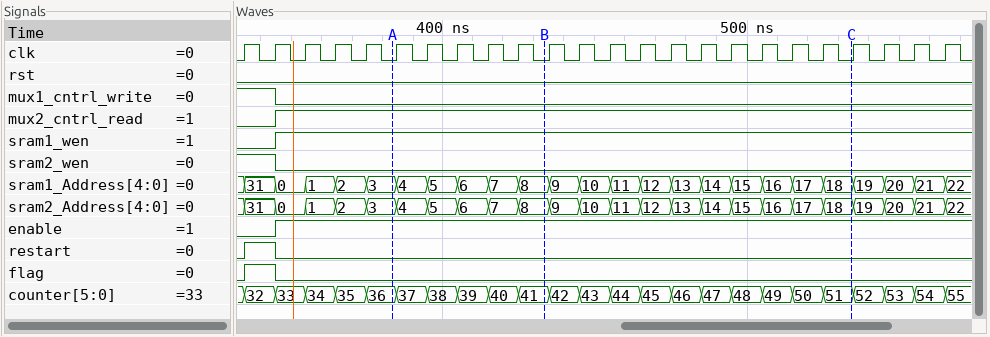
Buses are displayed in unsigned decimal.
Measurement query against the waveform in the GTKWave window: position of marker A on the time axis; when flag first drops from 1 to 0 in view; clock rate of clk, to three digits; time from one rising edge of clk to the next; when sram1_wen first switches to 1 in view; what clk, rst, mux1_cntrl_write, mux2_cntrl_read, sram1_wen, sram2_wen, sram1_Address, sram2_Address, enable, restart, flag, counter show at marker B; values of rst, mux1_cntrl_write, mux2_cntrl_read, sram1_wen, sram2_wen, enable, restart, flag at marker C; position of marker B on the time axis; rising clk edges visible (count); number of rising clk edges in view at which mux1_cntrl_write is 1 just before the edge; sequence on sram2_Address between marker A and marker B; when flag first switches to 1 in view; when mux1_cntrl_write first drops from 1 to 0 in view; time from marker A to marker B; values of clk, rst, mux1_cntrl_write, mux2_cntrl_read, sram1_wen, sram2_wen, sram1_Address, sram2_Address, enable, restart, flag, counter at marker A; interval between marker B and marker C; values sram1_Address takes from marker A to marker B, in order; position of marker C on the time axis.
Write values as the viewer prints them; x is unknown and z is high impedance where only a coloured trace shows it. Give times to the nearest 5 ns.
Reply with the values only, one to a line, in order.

385 ns
345 ns
100 MHz
10 ns
345 ns
clk=0, rst=0, mux1_cntrl_write=0, mux2_cntrl_read=1, sram1_wen=1, sram2_wen=0, sram1_Address=8, sram2_Address=8, enable=1, restart=0, flag=0, counter=41
rst=0, mux1_cntrl_write=0, mux2_cntrl_read=1, sram1_wen=1, sram2_wen=0, enable=1, restart=0, flag=0
435 ns
24
2
3, 4, 5, 6, 7, 8
335 ns
345 ns
50 ns
clk=0, rst=0, mux1_cntrl_write=0, mux2_cntrl_read=1, sram1_wen=1, sram2_wen=0, sram1_Address=3, sram2_Address=3, enable=1, restart=0, flag=0, counter=36
100 ns
3, 4, 5, 6, 7, 8
535 ns
